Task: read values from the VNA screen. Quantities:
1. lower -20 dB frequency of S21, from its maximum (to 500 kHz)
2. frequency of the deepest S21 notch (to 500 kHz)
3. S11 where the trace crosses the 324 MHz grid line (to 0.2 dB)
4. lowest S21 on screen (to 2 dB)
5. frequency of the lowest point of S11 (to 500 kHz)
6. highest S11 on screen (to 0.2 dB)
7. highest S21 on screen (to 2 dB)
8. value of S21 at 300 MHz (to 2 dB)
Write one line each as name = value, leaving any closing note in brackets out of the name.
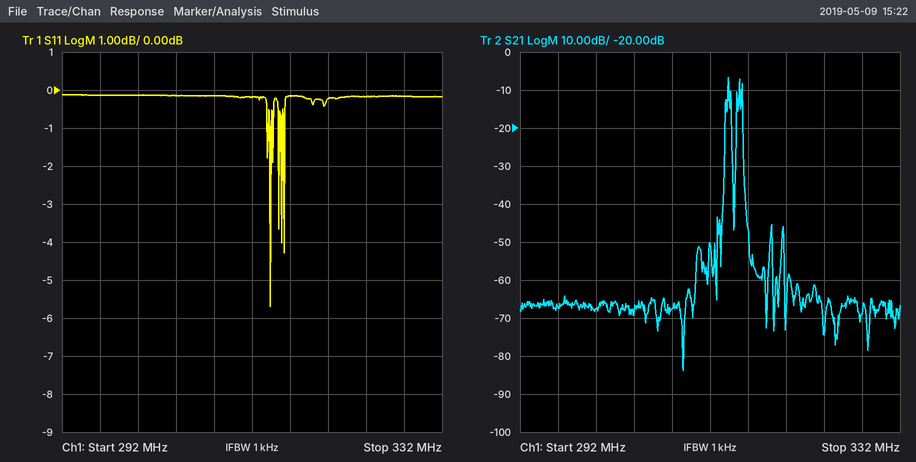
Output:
lower -20 dB frequency of S21, from its maximum = 313.5 MHz
frequency of the deepest S21 notch = 309.0 MHz
S11 where the trace crosses the 324 MHz grid line = -0.2 dB
lowest S21 on screen = -84 dB
frequency of the lowest point of S11 = 314.0 MHz
highest S11 on screen = -0.2 dB
highest S21 on screen = -6 dB
value of S21 at 300 MHz = -68 dB
